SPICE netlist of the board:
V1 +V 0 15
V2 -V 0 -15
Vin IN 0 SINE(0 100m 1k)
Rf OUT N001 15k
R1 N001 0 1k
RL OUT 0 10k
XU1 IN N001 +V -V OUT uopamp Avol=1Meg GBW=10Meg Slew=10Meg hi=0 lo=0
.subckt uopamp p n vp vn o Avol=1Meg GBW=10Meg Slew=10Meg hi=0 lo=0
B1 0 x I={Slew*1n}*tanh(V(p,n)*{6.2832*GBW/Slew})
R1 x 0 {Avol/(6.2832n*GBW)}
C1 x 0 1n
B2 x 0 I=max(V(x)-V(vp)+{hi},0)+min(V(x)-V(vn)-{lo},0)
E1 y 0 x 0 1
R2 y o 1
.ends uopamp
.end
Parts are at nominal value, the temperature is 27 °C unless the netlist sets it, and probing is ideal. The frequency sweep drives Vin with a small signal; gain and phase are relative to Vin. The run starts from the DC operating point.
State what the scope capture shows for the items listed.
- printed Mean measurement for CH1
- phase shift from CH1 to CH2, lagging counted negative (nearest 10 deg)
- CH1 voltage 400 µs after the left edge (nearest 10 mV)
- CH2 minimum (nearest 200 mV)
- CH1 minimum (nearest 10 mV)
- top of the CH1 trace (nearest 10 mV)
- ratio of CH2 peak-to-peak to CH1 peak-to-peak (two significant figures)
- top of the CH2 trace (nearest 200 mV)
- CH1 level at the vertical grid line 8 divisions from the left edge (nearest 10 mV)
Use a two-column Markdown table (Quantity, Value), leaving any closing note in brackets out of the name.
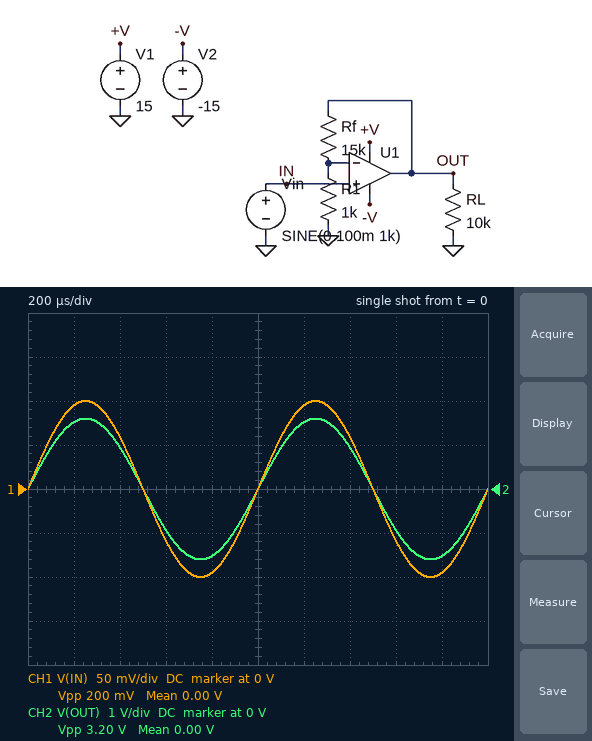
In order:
| Quantity | Value |
|---|---|
| printed Mean measurement for CH1 | 0.00 V |
| phase shift from CH1 to CH2, lagging counted negative | 0 deg |
| CH1 voltage 400 µs after the left edge | 60 mV |
| CH2 minimum | -1.6 V |
| CH1 minimum | -100 mV |
| top of the CH1 trace | 100 mV |
| ratio of CH2 peak-to-peak to CH1 peak-to-peak | 16 |
| top of the CH2 trace | 1.6 V |
| CH1 level at the vertical grid line 8 divisions from the left edge | -60 mV |
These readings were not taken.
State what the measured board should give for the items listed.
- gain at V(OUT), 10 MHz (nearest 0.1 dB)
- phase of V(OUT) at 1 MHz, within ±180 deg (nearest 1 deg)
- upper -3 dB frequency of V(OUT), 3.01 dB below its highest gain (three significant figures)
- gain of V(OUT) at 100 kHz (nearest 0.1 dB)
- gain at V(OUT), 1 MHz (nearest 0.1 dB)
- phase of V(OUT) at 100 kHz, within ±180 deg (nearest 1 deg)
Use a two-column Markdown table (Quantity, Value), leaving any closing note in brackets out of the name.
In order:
| Quantity | Value |
|---|---|
| gain at V(OUT), 10 MHz | 0 dB |
| phase of V(OUT) at 1 MHz, within ±180 deg | -58 deg |
| upper -3 dB frequency of V(OUT), 3.01 dB below its highest gain | 625 kHz |
| gain of V(OUT) at 100 kHz | 24.0 dB |
| gain at V(OUT), 1 MHz | 18.6 dB |
| phase of V(OUT) at 100 kHz, within ±180 deg | -9 deg |
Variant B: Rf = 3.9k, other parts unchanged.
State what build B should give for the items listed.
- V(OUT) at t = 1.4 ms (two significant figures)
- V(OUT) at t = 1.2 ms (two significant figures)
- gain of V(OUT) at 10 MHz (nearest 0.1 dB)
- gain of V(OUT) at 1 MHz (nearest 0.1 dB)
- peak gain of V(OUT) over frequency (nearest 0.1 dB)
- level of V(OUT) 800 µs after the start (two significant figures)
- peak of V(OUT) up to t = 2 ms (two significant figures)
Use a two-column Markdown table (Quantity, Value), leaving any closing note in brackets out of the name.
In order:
| Quantity | Value |
|---|---|
| V(OUT) at t = 1.4 ms | 290 mV |
| V(OUT) at t = 1.2 ms | 470 mV |
| gain of V(OUT) at 10 MHz | -0.2 dB |
| gain of V(OUT) at 1 MHz | 12.9 dB |
| peak gain of V(OUT) over frequency | 13.8 dB |
| level of V(OUT) 800 µs after the start | -470 mV |
| peak of V(OUT) up to t = 2 ms | 490 mV |
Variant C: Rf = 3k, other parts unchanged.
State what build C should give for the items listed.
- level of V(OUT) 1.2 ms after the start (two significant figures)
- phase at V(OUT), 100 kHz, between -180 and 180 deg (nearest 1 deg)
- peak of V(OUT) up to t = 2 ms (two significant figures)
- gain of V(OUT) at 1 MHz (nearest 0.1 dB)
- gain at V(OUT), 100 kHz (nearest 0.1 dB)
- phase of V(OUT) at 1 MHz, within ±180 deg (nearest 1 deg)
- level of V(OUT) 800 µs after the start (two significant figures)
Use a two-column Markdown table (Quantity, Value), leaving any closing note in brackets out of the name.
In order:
| Quantity | Value |
|---|---|
| level of V(OUT) 1.2 ms after the start | 380 mV |
| phase at V(OUT), 100 kHz, between -180 and 180 deg | -2 deg |
| peak of V(OUT) up to t = 2 ms | 400 mV |
| gain of V(OUT) at 1 MHz | 11.4 dB |
| gain at V(OUT), 100 kHz | 12.0 dB |
| phase of V(OUT) at 1 MHz, within ±180 deg | -22 deg |
| level of V(OUT) 800 µs after the start | -380 mV |
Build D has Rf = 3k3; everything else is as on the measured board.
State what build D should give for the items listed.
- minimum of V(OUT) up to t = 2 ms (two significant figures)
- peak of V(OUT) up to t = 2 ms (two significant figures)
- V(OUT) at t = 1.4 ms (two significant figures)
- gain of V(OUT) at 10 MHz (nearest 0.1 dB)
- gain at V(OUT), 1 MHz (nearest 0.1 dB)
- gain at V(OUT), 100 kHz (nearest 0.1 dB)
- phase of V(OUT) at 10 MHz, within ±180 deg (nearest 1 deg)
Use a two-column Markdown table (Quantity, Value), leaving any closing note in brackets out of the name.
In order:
| Quantity | Value |
|---|---|
| minimum of V(OUT) up to t = 2 ms | -430 mV |
| peak of V(OUT) up to t = 2 ms | 430 mV |
| V(OUT) at t = 1.4 ms | 250 mV |
| gain of V(OUT) at 10 MHz | -0.2 dB |
| gain at V(OUT), 1 MHz | 11.9 dB |
| gain at V(OUT), 100 kHz | 12.7 dB |
| phase of V(OUT) at 10 MHz, within ±180 deg | -77 deg |
